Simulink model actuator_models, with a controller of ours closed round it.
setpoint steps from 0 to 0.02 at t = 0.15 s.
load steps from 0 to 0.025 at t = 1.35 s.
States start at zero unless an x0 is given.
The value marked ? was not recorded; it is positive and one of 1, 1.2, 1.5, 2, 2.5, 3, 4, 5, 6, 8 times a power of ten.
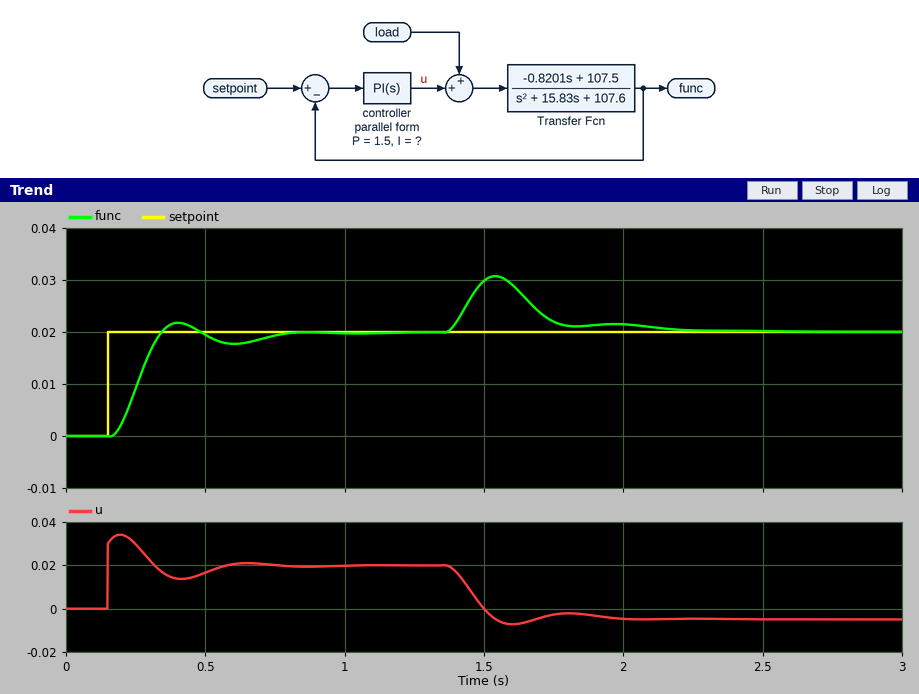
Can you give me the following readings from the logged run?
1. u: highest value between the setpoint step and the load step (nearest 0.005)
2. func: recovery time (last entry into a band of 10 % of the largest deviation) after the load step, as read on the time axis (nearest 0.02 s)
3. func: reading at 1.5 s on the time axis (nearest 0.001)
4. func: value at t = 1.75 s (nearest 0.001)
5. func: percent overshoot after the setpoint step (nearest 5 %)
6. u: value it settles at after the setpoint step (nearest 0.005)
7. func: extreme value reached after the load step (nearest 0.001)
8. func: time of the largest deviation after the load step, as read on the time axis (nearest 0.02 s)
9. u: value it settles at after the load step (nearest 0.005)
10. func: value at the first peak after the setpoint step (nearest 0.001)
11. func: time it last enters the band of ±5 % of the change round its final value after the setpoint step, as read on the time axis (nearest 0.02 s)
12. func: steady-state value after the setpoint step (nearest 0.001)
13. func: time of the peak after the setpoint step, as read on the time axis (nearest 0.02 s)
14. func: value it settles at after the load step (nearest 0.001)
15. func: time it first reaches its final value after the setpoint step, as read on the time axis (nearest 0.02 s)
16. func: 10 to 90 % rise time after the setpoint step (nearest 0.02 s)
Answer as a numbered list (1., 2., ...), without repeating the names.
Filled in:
1. 0.035
2. 2.08 s
3. 0.030
4. 0.022
5. 10 %
6. 0.020
7. 0.031
8. 1.54 s
9. -0.005
10. 0.022
11. 0.72 s
12. 0.020
13. 0.40 s
14. 0.020
15. 0.34 s
16. 0.12 s
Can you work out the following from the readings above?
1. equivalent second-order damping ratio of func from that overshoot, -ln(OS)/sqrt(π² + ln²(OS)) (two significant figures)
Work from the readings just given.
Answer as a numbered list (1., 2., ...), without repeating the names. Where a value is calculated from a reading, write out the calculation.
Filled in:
1. ln(0.1) = -2.303; 2.303 / sqrt(9.870 + 5.302) = 0.59
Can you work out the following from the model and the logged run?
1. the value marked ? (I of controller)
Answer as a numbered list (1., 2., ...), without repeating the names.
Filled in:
1. 8
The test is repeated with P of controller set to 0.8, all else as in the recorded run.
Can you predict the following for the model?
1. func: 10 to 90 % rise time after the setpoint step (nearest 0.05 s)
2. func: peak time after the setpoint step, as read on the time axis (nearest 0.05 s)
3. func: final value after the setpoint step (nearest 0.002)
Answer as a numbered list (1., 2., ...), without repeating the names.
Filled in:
1. 0.15 s
2. 0.50 s
3. 0.020
